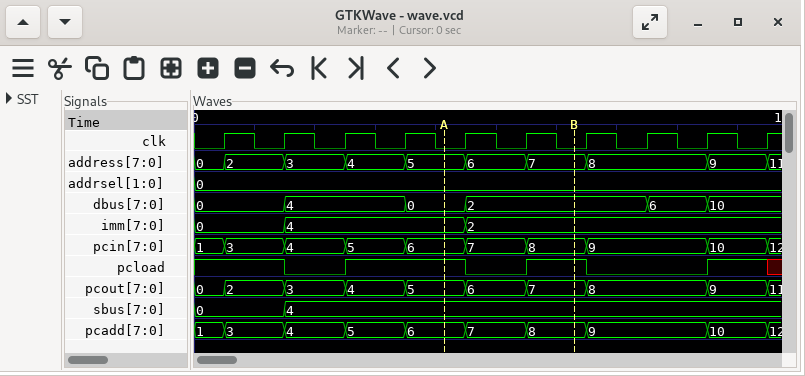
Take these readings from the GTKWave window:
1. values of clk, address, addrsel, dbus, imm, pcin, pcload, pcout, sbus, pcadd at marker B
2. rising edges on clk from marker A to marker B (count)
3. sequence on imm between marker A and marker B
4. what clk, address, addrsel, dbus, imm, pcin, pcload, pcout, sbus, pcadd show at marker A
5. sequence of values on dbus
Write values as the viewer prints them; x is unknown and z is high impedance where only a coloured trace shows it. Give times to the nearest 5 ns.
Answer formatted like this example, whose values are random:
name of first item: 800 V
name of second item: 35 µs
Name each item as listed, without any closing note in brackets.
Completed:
values of clk, address, addrsel, dbus, imm, pcin, pcload, pcout, sbus, pcadd at marker B: clk=0, address=7, addrsel=0, dbus=2, imm=2, pcin=8, pcload=1, pcout=7, sbus=4, pcadd=8
rising edges on clk from marker A to marker B: 2
sequence on imm between marker A and marker B: 4, 2
what clk, address, addrsel, dbus, imm, pcin, pcload, pcout, sbus, pcadd show at marker A: clk=0, address=5, addrsel=0, dbus=0, imm=4, pcin=6, pcload=1, pcout=5, sbus=4, pcadd=6
sequence of values on dbus: 0, 4, 0, 2, 6, 10
